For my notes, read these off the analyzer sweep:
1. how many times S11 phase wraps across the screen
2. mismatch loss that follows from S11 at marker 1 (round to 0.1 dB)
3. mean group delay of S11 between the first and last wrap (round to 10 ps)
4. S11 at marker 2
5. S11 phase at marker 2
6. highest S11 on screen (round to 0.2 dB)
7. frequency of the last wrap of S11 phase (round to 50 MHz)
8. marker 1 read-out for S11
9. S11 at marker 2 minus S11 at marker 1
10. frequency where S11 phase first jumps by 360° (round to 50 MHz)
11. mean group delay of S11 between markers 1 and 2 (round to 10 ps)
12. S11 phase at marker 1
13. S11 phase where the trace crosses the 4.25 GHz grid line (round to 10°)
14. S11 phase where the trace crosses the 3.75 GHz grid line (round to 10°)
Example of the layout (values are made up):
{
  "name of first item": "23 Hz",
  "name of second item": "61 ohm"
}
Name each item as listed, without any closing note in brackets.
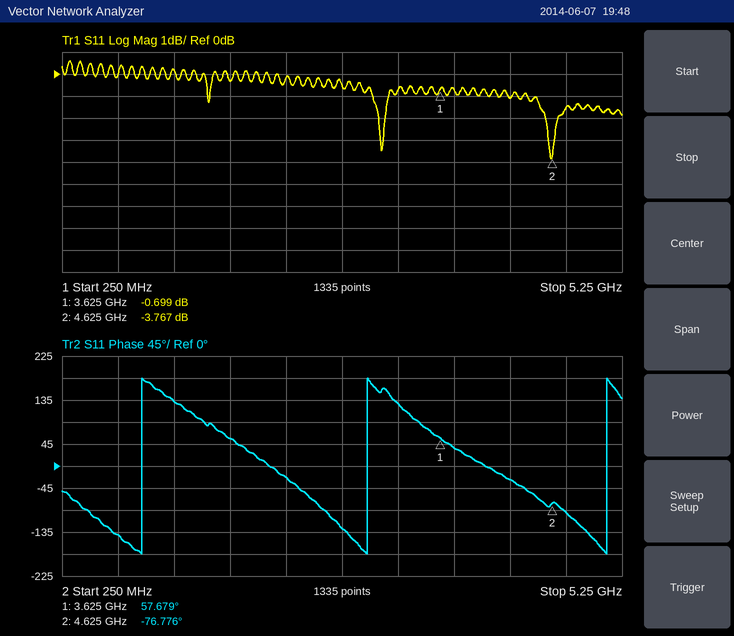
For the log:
{
  "how many times S11 phase wraps across the screen": "3",
  "mismatch loss that follows from S11 at marker 1": "8.3 dB",
  "mean group delay of S11 between the first and last wrap": "480 ps",
  "S11 at marker 2": "-3.767 dB",
  "S11 phase at marker 2": "-76.776°",
  "highest S11 on screen": "0.6 dB",
  "frequency of the last wrap of S11 phase": "5.10 GHz",
  "marker 1 read-out for S11": "-0.699 dB",
  "S11 at marker 2 minus S11 at marker 1": "-3.068 dB",
  "frequency where S11 phase first jumps by 360°": "950 MHz",
  "mean group delay of S11 between markers 1 and 2": "370 ps",
  "S11 phase at marker 1": "57.679°",
  "S11 phase where the trace crosses the 4.25 GHz grid line": "-30°",
  "S11 phase where the trace crosses the 3.75 GHz grid line": "40°"
}
